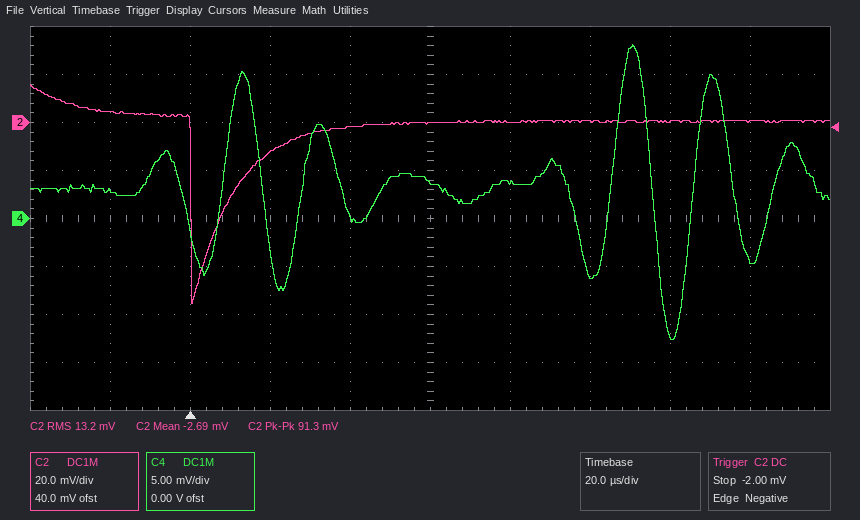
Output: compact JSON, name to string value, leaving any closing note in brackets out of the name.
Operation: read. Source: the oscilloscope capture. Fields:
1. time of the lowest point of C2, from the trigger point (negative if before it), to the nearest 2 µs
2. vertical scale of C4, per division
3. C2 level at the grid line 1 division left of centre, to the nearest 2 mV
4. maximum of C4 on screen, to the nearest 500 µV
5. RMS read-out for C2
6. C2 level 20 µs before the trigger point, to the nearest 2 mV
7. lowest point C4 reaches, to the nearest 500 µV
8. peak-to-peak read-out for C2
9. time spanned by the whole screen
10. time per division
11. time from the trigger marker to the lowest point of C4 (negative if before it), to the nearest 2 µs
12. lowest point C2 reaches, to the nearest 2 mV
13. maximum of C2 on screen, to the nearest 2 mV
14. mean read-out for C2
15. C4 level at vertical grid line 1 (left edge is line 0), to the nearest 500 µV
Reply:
{"time of the lowest point of C2, from the trigger point (negative if before it), to the nearest 2 µs": "0 µs", "vertical scale of C4, per division": "5 mV", "C2 level at the grid line 1 division left of centre, to the nearest 2 mV": "-2 mV", "maximum of C4 on screen, to the nearest 500 µV": "18.0 mV", "RMS read-out for C2": "13.2 mV", "C2 level 20 µs before the trigger point, to the nearest 2 mV": "4 mV", "lowest point C4 reaches, to the nearest 500 µV": "-12.5 mV", "peak-to-peak read-out for C2": "91.3 mV", "time spanned by the whole screen": "200 µs", "time per division": "20 µs", "time from the trigger marker to the lowest point of C4 (negative if before it), to the nearest 2 µs": "+120 µs", "lowest point C2 reaches, to the nearest 2 mV": "-76 mV", "maximum of C2 on screen, to the nearest 2 mV": "16 mV", "mean read-out for C2": "-2.69 mV", "C4 level at vertical grid line 1 (left edge is line 0), to the nearest 500 µV": "3.0 mV"}
